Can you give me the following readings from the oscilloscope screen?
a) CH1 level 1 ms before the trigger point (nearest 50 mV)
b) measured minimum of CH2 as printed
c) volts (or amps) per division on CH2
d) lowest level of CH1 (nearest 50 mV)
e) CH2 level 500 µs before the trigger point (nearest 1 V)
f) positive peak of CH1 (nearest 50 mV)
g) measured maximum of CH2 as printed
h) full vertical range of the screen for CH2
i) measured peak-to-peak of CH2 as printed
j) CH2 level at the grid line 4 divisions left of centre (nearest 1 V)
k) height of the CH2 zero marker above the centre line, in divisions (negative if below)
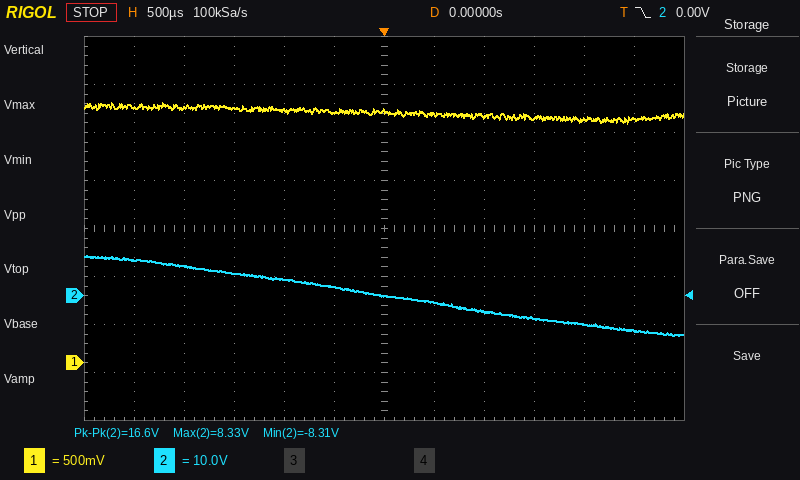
2.65 V
-8.31 V
10 V
2.50 V
2 V
2.70 V
8.33 V
80 V
16.6 V
6 V
-1.4 div
